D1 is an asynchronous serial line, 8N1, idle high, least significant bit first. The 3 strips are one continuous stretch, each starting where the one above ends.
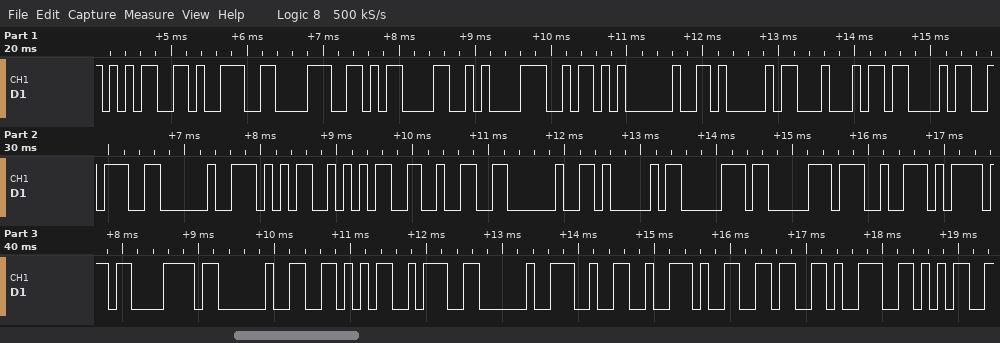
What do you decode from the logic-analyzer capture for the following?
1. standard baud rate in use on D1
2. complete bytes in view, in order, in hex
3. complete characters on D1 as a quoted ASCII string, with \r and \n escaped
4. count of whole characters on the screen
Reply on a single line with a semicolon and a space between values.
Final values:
9600 baud; 0x35 0x39 0x38 0x0D 0x0A 0x5A 0x20 0x41 0x44 0x43 0x3A 0x20 0x35 0x35 0x32 0x20 0x41 0x70 0x70 0x72 0x6F 0x78 0x20 0x56 0x3A 0x20 0x32 0x2E 0x36 0x39 0x35; "598\r\nZ ADC: 552 Approx V: 2.695"; 31
